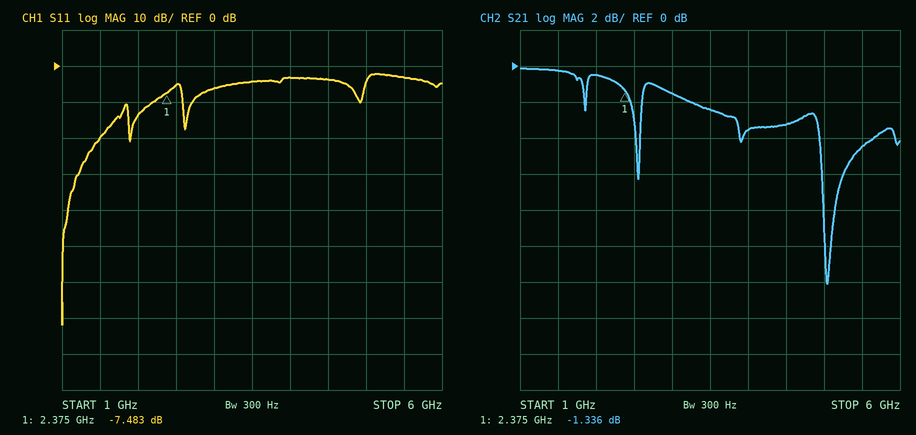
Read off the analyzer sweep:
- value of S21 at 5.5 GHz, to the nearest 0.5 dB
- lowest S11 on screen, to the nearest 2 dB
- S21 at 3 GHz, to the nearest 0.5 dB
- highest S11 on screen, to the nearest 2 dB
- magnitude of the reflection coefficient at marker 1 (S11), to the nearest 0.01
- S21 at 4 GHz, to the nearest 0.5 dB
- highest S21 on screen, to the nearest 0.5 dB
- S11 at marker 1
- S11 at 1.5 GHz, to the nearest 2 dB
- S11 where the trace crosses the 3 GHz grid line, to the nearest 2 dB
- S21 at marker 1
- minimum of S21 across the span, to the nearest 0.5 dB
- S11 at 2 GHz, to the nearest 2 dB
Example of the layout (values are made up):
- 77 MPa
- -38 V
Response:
- -4.5 dB
- -72 dB
- -1.5 dB
- -2 dB
- 0.42
- -3.5 dB
- 0.0 dB
- -7.483 dB
- -20 dB
- -6 dB
- -1.336 dB
- -12.0 dB
- -14 dB
